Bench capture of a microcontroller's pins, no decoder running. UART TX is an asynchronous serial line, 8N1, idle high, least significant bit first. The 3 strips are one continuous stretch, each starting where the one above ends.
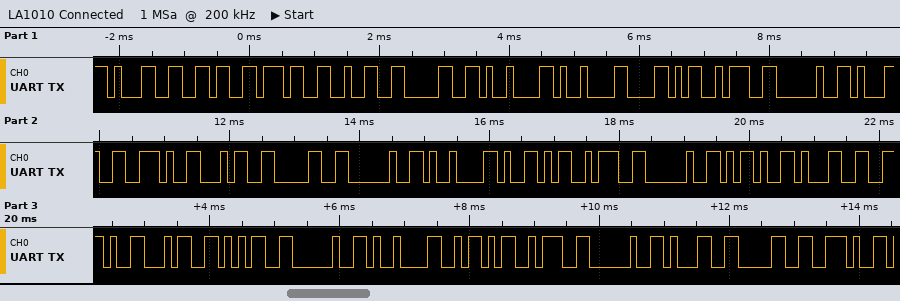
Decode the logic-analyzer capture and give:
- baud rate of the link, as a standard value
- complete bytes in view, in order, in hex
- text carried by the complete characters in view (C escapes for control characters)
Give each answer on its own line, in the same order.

9600 baud
0x31 0x36 0x37 0x32 0x30 0x09 0x09 0x58 0x3A 0x20 0x31 0x2E 0x34 0x30 0x20 0x09 0x59 0x3A 0x20 0x2D 0x31 0x2E 0x34 0x35 0x20 0x09 0x5A 0x3A 0x20 0x31 0x30 0x2E
"16720\t\tX: 1.40 \tY: -1.45 \tZ: 10."
